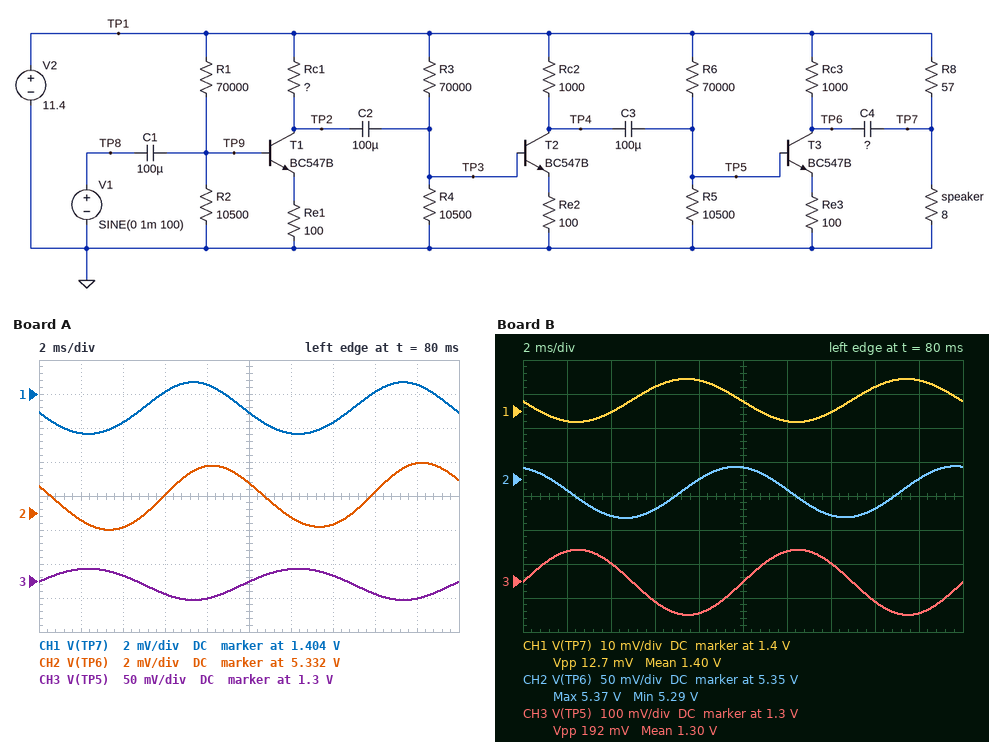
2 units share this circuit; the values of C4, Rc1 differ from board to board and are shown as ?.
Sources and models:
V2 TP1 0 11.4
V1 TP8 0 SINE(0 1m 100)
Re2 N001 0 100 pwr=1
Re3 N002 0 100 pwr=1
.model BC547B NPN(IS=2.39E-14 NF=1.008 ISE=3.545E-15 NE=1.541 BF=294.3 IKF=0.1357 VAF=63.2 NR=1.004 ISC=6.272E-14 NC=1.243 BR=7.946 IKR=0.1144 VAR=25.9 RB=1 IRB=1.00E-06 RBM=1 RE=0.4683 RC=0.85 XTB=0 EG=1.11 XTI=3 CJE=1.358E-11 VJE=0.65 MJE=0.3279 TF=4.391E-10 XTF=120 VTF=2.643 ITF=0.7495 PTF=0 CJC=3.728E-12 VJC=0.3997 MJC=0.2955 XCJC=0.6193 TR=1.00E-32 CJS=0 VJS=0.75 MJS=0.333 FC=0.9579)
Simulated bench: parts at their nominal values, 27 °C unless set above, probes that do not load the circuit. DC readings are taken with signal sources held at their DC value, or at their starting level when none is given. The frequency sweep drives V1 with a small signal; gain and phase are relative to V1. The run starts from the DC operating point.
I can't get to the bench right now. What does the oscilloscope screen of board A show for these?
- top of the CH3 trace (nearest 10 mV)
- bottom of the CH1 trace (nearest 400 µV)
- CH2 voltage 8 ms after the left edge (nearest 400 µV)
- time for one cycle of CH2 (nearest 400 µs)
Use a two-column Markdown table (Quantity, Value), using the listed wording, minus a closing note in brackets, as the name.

| Quantity | Value |
|---|---|
| top of the CH3 trace | 1.32 V |
| bottom of the CH1 trace | 1.4016 V |
| CH2 voltage 8 ms after the left edge | 5.3348 V |
| time for one cycle of CH2 | 10.0 ms |
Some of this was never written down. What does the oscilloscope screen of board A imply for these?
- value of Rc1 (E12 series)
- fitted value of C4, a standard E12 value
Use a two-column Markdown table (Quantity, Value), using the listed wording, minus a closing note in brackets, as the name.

| Quantity | Value |
|---|---|
| value of Rc1 | 3.3 kΩ |
| fitted value of C4, a standard E12 value | 330 µF |
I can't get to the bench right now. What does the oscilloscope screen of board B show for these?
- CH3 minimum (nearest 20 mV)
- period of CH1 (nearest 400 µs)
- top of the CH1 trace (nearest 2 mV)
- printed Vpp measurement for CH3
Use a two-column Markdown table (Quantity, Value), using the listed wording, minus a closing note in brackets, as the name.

| Quantity | Value |
|---|---|
| CH3 minimum | 1.20 V |
| period of CH1 | 10.0 ms |
| top of the CH1 trace | 1.410 V |
| printed Vpp measurement for CH3 | 192 mV |
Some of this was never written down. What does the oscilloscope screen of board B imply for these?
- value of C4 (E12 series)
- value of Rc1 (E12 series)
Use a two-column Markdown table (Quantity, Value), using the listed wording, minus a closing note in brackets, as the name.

| Quantity | Value |
|---|---|
| value of C4 | 39 µF |
| value of Rc1 | 1.5 kΩ |
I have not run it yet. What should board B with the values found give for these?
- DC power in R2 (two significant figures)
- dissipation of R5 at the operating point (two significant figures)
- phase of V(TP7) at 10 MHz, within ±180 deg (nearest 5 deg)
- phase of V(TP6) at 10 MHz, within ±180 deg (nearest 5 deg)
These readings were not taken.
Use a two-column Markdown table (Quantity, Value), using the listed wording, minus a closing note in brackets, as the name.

| Quantity | Value |
|---|---|
| DC power in R2 | 160 µW |
| dissipation of R5 at the operating point | 160 µW |
| phase of V(TP7) at 10 MHz, within ±180 deg | 90 deg |
| phase of V(TP6) at 10 MHz, within ±180 deg | 90 deg |
